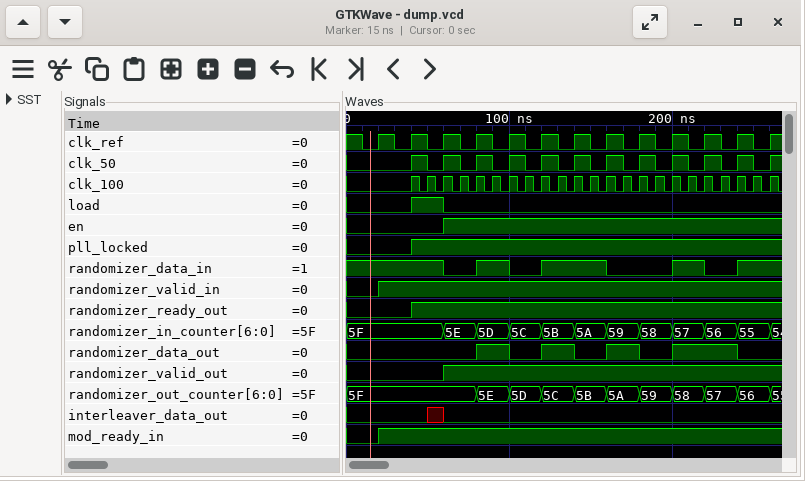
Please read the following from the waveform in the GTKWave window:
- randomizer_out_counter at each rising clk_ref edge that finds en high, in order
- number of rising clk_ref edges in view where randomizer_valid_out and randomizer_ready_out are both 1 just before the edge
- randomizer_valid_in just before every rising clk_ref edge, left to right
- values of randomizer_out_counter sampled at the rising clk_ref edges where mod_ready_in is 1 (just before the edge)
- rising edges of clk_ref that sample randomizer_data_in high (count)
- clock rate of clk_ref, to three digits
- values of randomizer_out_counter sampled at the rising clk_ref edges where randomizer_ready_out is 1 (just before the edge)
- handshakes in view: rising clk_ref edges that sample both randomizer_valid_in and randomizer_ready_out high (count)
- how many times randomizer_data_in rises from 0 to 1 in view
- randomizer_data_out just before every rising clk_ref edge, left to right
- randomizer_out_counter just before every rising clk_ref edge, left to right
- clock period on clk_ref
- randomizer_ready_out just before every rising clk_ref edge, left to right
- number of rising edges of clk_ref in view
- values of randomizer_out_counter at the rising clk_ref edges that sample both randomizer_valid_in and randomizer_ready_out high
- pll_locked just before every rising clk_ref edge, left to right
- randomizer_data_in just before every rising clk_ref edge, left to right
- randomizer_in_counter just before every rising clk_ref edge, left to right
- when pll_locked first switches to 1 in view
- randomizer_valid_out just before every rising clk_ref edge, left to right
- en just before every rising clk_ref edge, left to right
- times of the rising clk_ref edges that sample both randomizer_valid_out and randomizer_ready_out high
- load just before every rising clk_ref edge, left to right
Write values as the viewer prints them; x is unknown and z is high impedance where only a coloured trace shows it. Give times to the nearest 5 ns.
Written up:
5F, 5E, 5D, 5C, 5B, 5A, 59, 58, 57, 56
10
0 1 1 1 1 1 1 1 1 1 1 1 1
5F, 5F, 5F, 5E, 5D, 5C, 5B, 5A, 59, 58, 57, 56
8
50.0 MHz
5F, 5F, 5E, 5D, 5C, 5B, 5A, 59, 58, 57, 56
11
4
0 0 0 0 1 0 1 0 1 0 1 1 0
5F, 5F, 5F, 5F, 5E, 5D, 5C, 5B, 5A, 59, 58, 57, 56
20 ns
0 0 1 1 1 1 1 1 1 1 1 1 1
13
5F, 5F, 5E, 5D, 5C, 5B, 5A, 59, 58, 57, 56
0 0 1 1 1 1 1 1 1 1 1 1 1
1 1 1 0 1 0 1 1 0 0 1 0 1
5F, 5F, 5F, 5E, 5D, 5C, 5B, 5A, 59, 58, 57, 56, 55
40 ns
0 0 0 1 1 1 1 1 1 1 1 1 1
0 0 0 1 1 1 1 1 1 1 1 1 1
80 ns, 100 ns, 120 ns, 140 ns, 160 ns, 180 ns, 200 ns, 220 ns, 240 ns, 260 ns
0 0 1 0 0 0 0 0 0 0 0 0 0
